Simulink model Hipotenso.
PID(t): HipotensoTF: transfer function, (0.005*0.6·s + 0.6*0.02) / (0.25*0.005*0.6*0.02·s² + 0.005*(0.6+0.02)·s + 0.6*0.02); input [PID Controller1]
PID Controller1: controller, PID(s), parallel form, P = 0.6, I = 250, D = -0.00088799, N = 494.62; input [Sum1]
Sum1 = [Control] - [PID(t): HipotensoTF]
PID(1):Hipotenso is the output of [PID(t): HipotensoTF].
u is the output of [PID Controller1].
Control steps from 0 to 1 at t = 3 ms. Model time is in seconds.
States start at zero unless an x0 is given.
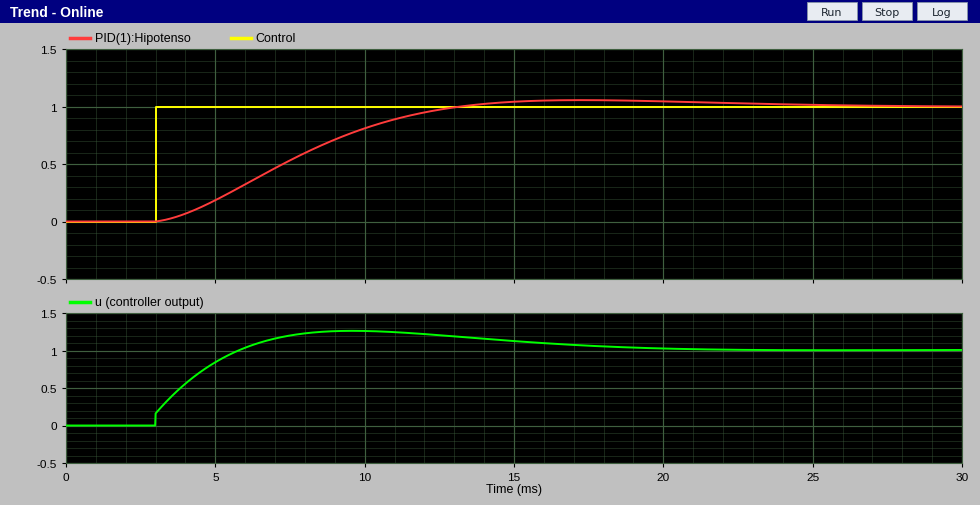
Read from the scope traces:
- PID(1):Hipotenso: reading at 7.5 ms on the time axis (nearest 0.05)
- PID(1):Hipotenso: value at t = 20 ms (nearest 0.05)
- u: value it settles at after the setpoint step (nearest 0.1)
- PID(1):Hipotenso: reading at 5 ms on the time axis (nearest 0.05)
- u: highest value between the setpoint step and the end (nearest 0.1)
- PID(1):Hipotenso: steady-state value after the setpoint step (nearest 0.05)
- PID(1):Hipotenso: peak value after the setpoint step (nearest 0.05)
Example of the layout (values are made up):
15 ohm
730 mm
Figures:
0.55
1.05
1.0
0.20
1.3
1.00
1.05
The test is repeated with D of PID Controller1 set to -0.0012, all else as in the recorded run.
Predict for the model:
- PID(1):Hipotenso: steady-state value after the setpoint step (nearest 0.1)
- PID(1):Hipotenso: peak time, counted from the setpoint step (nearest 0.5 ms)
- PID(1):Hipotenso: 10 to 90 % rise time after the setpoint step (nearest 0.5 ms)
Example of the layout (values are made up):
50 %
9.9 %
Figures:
1.0
13.5 ms
6.5 ms
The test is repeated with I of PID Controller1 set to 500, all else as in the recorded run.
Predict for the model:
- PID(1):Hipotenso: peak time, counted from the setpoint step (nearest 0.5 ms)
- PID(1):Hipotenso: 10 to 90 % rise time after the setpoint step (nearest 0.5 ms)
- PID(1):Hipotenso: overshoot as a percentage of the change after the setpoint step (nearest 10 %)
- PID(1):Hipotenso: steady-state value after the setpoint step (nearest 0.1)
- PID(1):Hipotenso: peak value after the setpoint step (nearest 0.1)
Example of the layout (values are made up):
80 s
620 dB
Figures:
9.5 ms
4.0 ms
20 %
1.0
1.2
